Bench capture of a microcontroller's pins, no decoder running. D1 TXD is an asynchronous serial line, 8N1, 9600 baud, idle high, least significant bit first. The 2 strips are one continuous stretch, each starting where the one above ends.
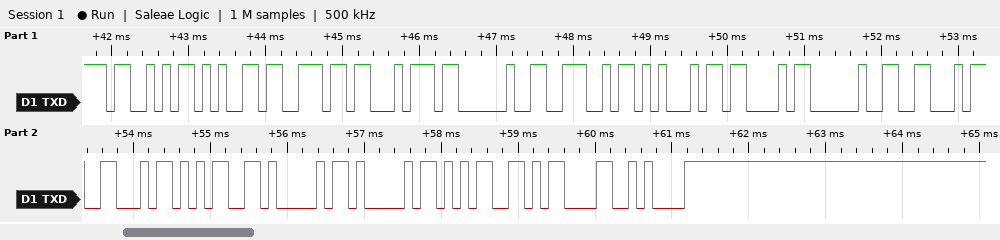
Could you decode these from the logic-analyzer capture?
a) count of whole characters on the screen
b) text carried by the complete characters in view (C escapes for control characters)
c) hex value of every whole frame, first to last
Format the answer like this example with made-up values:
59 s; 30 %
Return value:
17; "Sent NEC FF5AA5\r\n"; 53 65 6E 74 20 4E 45 43 20 46 46 35 41 41 35 0D 0A
